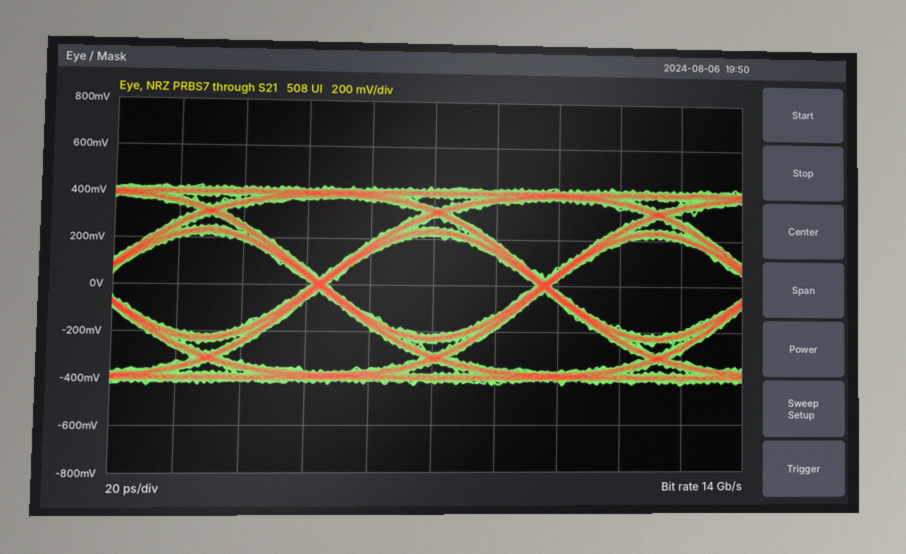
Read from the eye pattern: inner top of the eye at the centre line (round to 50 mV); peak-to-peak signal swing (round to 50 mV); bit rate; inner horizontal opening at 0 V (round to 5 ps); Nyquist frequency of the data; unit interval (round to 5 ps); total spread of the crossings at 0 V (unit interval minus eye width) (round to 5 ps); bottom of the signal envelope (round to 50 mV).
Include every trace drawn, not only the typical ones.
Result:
200 mV
850 mV
14 Gb/s
65 ps
7 GHz
70 ps
5 ps
-450 mV
